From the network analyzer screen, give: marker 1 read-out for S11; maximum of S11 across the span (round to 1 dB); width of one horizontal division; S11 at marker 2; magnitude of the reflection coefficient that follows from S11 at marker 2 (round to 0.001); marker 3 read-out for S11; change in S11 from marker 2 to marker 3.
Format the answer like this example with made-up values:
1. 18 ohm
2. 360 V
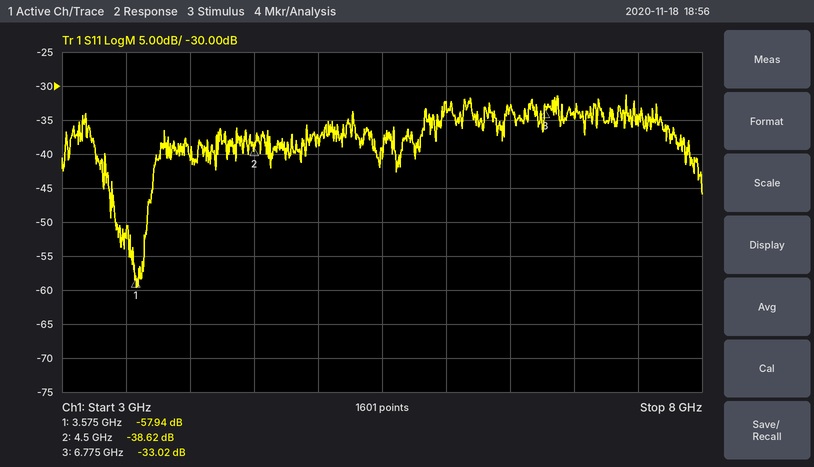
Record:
1. -57.94 dB
2. -31 dB
3. 500 MHz
4. -38.62 dB
5. 0.012
6. -33.02 dB
7. 5.60 dB
